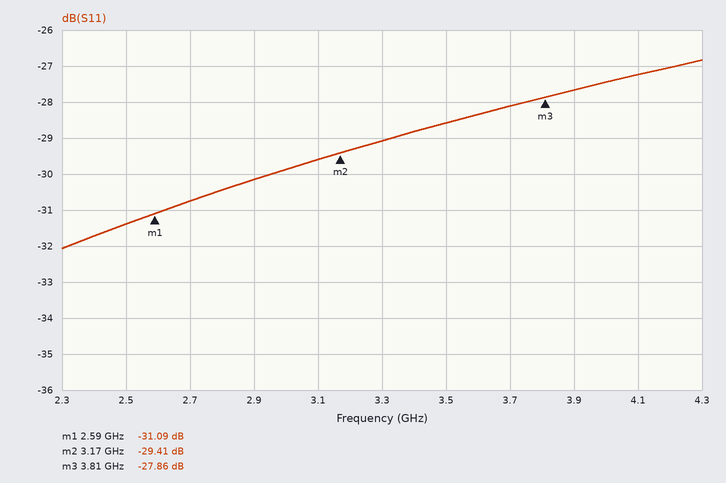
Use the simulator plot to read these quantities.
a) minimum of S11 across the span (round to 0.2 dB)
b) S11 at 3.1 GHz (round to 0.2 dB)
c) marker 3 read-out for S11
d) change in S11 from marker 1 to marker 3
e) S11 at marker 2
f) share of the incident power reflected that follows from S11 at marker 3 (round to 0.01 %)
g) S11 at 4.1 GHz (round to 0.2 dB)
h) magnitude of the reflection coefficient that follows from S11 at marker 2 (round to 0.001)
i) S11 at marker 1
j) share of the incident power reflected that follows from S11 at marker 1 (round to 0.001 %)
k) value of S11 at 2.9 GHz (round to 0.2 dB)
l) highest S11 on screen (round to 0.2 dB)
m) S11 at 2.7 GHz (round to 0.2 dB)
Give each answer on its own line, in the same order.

-32.0 dB
-29.6 dB
-27.86 dB
3.23 dB
-29.41 dB
0.16 %
-27.2 dB
0.034
-31.09 dB
0.078 %
-30.2 dB
-26.8 dB
-30.8 dB
